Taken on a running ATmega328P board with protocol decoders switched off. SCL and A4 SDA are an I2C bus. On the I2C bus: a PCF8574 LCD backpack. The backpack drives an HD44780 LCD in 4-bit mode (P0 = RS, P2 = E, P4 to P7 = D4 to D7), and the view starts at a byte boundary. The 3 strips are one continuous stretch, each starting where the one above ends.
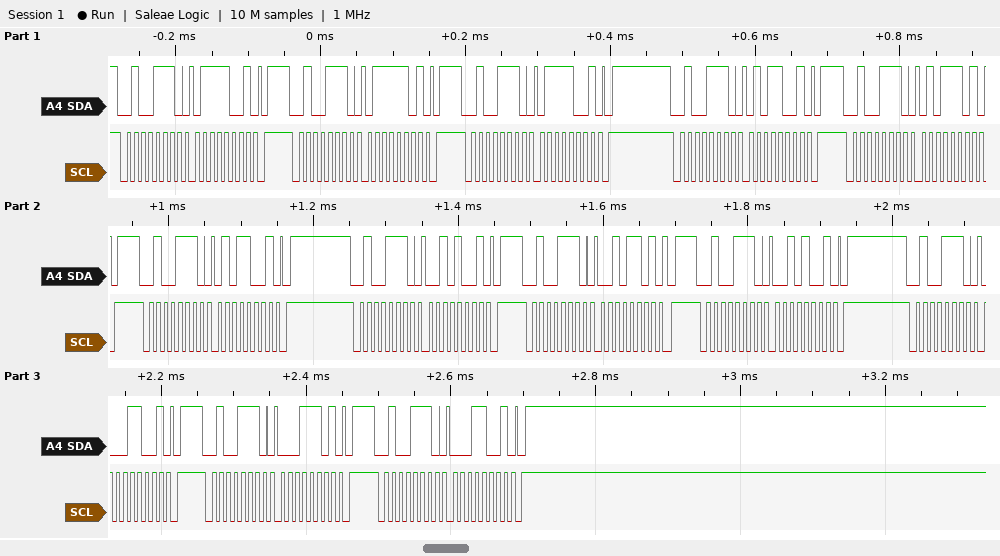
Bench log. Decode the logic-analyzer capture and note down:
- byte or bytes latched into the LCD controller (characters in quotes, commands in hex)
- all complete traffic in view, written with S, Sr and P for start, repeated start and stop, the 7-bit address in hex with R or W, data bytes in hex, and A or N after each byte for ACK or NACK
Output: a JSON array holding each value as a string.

["'u' '!'", "S 27W A 79 A P S 27W A 7D A P S 27W A 79 A P S 27W A 59 A P S 27W A 5D A P S 27W A 59 A P S 27W A 29 A P S 27W A 2D A P S 27W A 29 A P S 27W A 19 A P S 27W A 1D A P S 27W A 19 A P"]
